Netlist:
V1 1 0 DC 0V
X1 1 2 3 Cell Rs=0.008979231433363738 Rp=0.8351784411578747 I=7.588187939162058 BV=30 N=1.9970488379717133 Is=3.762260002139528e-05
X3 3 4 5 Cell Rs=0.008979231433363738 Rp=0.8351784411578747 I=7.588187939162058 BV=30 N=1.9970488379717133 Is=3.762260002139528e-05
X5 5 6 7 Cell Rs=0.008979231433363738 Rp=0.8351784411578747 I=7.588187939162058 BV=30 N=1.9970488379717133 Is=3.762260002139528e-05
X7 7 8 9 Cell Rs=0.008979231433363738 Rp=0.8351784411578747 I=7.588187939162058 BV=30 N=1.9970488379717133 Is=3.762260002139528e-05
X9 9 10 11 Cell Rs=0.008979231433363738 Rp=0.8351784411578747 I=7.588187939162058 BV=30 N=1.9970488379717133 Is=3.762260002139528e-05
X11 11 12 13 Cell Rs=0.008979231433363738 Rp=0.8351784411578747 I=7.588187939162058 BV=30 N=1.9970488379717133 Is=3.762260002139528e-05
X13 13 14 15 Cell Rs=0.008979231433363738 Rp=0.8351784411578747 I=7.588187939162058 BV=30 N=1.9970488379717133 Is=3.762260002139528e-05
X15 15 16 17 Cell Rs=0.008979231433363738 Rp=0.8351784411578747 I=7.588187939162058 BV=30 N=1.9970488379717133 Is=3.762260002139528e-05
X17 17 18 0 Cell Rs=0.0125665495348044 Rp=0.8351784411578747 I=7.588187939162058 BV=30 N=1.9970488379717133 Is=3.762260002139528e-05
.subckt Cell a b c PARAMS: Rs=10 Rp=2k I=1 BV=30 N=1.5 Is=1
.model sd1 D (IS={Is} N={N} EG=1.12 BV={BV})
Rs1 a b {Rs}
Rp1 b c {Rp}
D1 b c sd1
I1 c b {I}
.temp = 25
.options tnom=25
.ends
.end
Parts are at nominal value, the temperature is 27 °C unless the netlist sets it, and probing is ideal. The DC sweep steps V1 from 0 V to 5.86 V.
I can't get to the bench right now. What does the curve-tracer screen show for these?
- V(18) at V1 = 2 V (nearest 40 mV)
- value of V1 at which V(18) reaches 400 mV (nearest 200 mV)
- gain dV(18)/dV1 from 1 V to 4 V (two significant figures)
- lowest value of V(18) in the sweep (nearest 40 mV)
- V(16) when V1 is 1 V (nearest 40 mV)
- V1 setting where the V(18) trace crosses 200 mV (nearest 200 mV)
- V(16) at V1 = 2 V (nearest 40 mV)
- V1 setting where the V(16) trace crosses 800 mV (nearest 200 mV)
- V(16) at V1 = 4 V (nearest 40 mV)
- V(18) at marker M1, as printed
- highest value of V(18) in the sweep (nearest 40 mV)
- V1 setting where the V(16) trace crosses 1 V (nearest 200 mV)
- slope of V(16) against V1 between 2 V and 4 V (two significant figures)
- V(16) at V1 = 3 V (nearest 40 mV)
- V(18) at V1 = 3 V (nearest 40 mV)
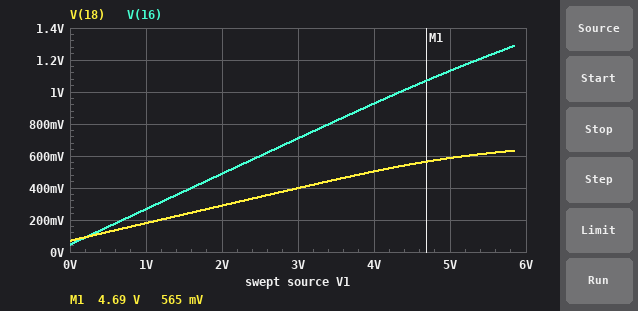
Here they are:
280 mV
3.0 V
0.11 V/V
80 mV
280 mV
1.2 V
480 mV
3.4 V
920 mV
565 mV
640 mV
4.4 V
0.22 V/V
720 mV
400 mV
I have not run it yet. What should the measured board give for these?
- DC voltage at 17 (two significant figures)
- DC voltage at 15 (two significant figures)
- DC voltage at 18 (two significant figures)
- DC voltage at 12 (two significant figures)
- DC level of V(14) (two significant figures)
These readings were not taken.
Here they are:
-24 mV
-21 mV
70 mV
52 mV
49 mV
